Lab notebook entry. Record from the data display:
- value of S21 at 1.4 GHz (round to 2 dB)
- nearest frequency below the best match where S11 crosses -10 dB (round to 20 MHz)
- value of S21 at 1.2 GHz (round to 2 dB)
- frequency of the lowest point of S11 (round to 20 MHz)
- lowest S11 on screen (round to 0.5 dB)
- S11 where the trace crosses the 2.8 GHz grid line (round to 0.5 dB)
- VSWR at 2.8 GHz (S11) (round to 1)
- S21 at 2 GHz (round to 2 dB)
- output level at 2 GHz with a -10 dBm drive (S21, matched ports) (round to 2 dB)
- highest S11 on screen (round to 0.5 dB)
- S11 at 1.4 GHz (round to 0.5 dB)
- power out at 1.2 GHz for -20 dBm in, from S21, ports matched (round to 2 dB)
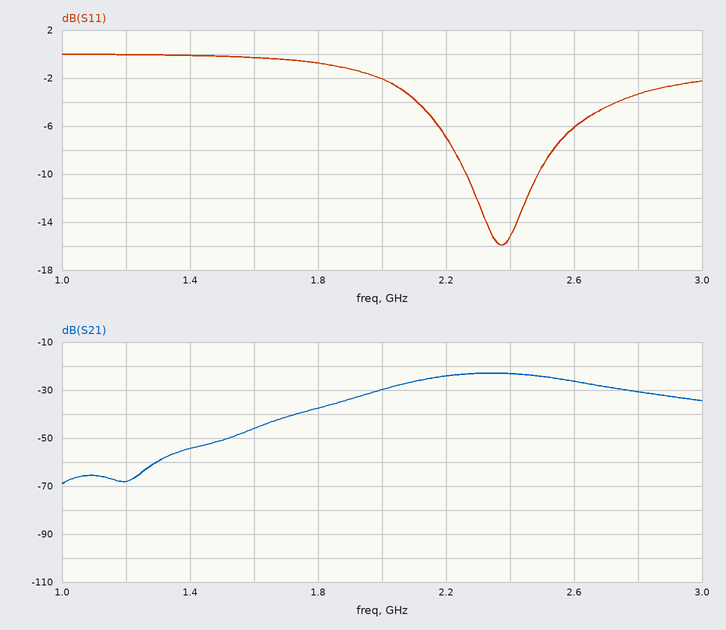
-54 dB
2.26 GHz
-68 dB
2.38 GHz
-16.0 dB
-3.5 dB
5
-30 dB
-40 dBm
0.0 dB
0.0 dB
-88 dBm
